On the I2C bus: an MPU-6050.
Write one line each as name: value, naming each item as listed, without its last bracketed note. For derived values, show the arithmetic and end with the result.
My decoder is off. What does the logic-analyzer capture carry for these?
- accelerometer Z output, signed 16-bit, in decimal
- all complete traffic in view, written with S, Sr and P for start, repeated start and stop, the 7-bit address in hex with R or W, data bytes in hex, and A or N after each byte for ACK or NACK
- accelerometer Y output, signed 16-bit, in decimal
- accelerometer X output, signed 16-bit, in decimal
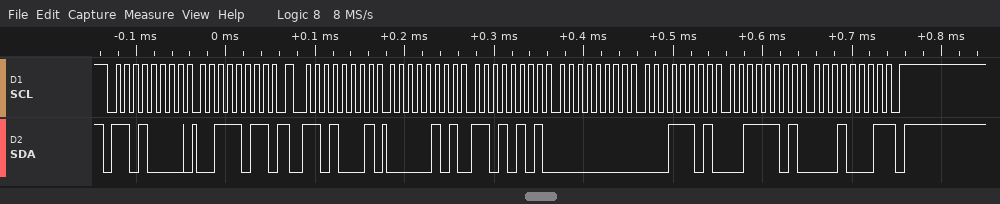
accelerometer Z output, signed 16-bit, in decimal: 0x3D11 = 15633
all complete traffic in view, written with S, Sr and P for start, repeated start and stop, the 7-bit address in hex with R or W, data bytes in hex, and A or N after each byte for ACK or NACK: S 68W A 3B A Sr 68R A 05 A D5 A 00 A 1D A 3D A 11 N P
accelerometer Y output, signed 16-bit, in decimal: 0x001D = 29
accelerometer X output, signed 16-bit, in decimal: 0x05D5 = 1493
